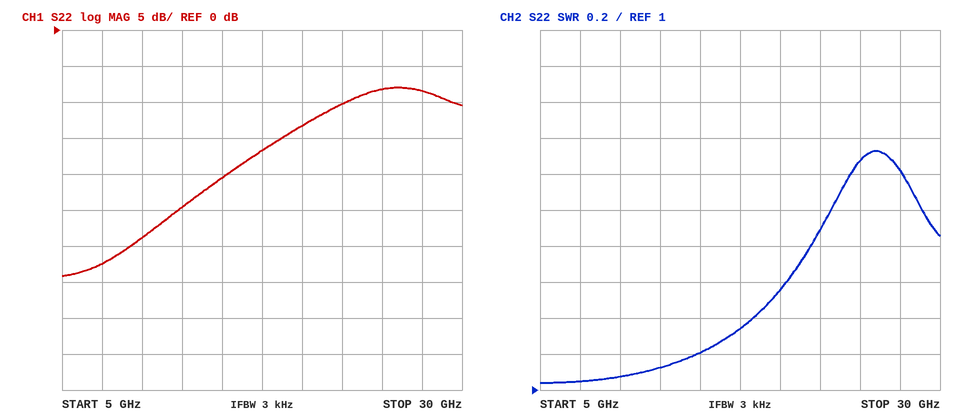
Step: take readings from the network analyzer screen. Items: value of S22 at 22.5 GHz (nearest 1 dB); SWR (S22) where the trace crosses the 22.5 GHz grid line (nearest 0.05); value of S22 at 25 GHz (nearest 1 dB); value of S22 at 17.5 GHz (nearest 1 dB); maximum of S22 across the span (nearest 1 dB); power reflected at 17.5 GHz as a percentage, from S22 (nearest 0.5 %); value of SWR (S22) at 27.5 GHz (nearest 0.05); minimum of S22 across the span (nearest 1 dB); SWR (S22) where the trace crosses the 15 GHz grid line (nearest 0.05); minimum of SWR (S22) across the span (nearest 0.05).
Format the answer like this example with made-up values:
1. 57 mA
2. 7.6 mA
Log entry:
1. -10 dB
2. 1.90
3. -8 dB
4. -17 dB
5. -8 dB
6. 2.0 %
7. 2.20
8. -34 dB
9. 1.20
10. 1.05
